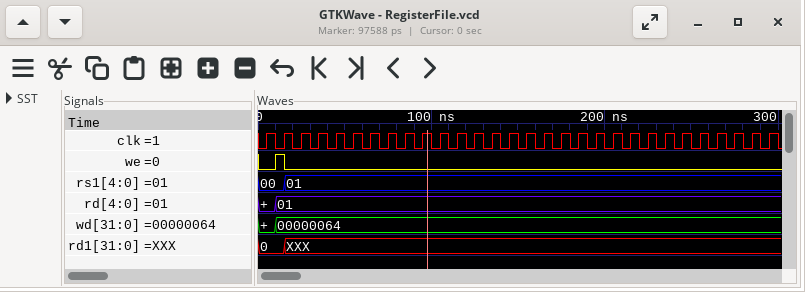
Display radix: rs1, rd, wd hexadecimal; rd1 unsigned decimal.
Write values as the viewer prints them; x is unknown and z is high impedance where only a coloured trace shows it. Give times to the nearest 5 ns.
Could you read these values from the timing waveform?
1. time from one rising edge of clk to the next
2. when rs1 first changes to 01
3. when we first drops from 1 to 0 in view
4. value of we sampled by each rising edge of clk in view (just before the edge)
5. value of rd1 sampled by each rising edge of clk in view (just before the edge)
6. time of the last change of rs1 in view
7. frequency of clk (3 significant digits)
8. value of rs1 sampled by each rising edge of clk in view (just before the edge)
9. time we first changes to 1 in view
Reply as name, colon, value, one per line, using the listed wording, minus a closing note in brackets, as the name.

time from one rising edge of clk to the next: 10 ns
when rs1 first changes to 01: 15 ns
when we first drops from 1 to 0 in view: 15 ns
value of we sampled by each rising edge of clk in view: 0 1 0 0 0 0 0 0 0 0 0 0 0 0 0 0 0 0 0 0 0 0 0 0 0 0 0 0 0 0
value of rd1 sampled by each rising edge of clk in view: 0, 0, XXX, XXX, XXX, XXX, XXX, XXX, XXX, XXX, XXX, XXX, XXX, XXX, XXX, XXX, XXX, XXX, XXX, XXX, XXX, XXX, XXX, XXX, XXX, XXX, XXX, XXX, XXX, XXX
time of the last change of rs1 in view: 15 ns
frequency of clk: 100 MHz
value of rs1 sampled by each rising edge of clk in view: 00, 00, 01, 01, 01, 01, 01, 01, 01, 01, 01, 01, 01, 01, 01, 01, 01, 01, 01, 01, 01, 01, 01, 01, 01, 01, 01, 01, 01, 01
time we first changes to 1 in view: 10 ns
